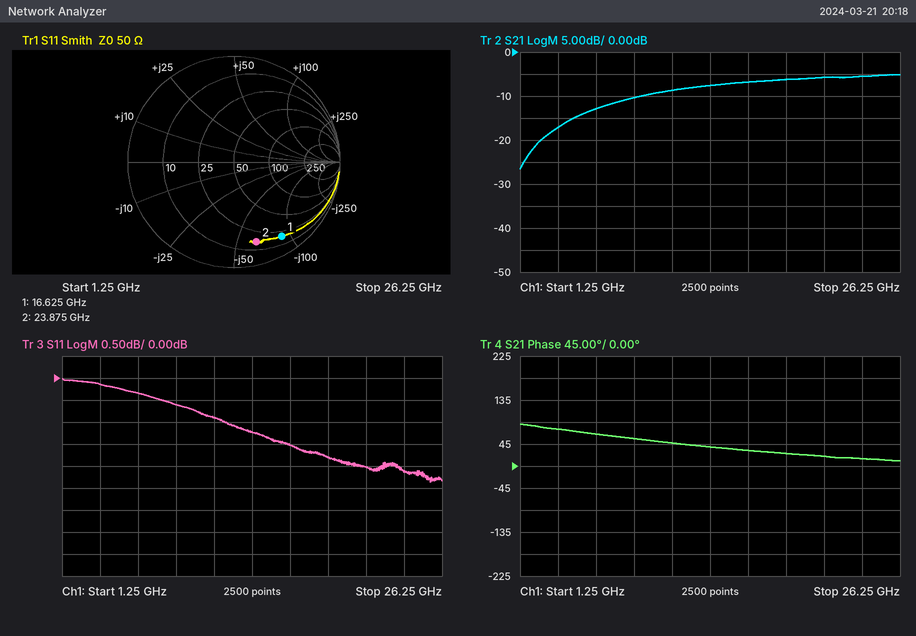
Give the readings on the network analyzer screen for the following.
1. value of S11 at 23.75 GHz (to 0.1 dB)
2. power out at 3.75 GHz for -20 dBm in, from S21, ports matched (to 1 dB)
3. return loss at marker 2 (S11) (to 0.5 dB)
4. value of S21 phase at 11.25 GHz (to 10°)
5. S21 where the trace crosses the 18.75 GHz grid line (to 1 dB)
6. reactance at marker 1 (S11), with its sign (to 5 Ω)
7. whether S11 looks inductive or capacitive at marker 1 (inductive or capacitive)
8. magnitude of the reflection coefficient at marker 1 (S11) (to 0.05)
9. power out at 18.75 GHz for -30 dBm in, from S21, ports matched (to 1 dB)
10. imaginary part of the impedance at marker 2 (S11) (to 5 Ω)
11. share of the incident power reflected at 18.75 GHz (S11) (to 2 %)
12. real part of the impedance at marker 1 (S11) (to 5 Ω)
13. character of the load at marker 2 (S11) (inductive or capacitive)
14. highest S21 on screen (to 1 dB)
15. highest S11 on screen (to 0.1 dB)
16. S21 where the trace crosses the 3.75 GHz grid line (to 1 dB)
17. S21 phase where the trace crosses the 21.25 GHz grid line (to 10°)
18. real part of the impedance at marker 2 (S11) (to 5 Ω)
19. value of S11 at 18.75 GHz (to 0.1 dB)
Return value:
-2.1 dB
-37 dBm
2.0 dB
50°
-6 dB
-90 Ω
capacitive
0.85
-36 dBm
-65 Ω
66 %
20 Ω
capacitive
-5 dB
0.0 dB
-17 dB
20°
15 Ω
-1.8 dB
